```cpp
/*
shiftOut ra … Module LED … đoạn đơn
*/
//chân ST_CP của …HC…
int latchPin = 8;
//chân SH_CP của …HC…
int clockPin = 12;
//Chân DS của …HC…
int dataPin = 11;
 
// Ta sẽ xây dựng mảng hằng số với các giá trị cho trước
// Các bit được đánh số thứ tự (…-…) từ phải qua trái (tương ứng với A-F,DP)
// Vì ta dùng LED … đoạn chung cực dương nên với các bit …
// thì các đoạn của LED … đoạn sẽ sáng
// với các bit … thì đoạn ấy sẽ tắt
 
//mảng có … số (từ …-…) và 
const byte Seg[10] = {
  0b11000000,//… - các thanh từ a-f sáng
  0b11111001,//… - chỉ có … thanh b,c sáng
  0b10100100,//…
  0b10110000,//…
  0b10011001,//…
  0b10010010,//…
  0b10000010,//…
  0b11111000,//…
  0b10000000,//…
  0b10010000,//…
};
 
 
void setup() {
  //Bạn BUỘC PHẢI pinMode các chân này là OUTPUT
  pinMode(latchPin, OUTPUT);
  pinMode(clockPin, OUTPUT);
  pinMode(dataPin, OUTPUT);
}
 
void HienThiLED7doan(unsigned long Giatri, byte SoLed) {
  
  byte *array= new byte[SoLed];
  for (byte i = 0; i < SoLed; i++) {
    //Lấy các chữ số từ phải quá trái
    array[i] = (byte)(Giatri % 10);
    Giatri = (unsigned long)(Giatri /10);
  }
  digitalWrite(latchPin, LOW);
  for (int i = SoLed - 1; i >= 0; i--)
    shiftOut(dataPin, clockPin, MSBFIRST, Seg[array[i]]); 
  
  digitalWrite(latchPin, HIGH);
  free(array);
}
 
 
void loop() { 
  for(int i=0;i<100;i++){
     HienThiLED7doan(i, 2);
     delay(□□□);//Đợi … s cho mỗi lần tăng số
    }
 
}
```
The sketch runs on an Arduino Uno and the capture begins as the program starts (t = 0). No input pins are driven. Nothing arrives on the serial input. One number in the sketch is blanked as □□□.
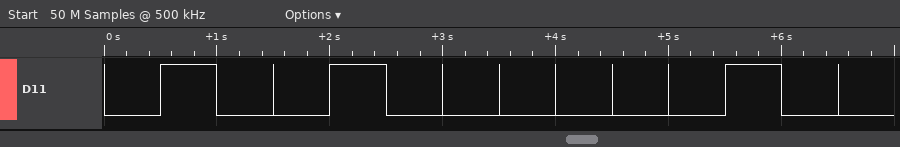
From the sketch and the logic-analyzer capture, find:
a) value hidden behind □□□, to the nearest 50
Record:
500
